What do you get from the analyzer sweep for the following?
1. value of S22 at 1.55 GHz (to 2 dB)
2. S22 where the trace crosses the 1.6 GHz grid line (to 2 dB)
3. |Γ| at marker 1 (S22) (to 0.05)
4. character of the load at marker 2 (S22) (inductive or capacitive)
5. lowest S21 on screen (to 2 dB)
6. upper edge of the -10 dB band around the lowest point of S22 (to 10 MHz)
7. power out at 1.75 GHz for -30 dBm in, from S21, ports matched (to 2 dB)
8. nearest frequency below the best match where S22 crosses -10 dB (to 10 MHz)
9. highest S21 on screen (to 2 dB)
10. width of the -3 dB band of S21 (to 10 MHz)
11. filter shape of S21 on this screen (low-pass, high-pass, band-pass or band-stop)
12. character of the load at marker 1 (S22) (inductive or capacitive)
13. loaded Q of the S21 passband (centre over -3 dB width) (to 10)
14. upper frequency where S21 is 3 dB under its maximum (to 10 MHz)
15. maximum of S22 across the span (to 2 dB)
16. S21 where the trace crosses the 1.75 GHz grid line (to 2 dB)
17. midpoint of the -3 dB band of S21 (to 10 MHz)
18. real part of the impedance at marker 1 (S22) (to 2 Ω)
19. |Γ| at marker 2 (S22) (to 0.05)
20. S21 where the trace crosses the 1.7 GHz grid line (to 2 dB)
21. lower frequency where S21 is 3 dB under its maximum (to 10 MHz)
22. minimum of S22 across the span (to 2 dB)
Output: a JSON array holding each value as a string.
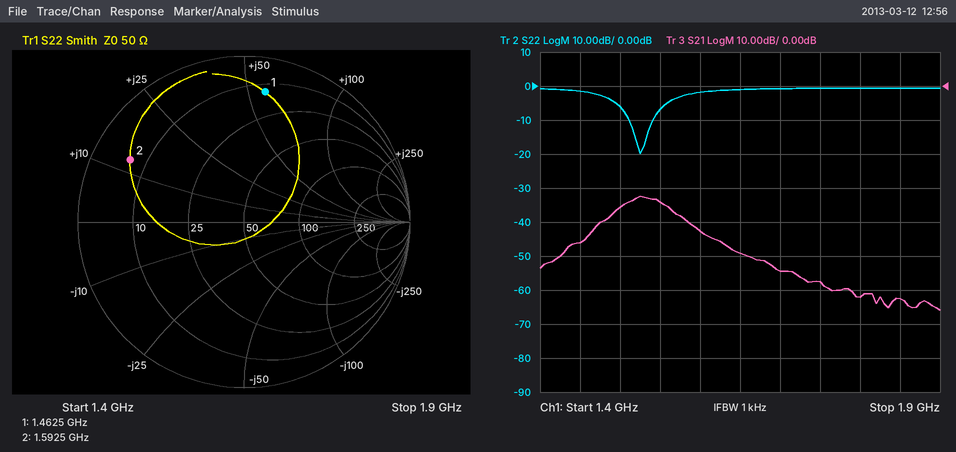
["-6 dB", "-2 dB", "0.80", "inductive", "-66 dB", "1.54 GHz", "-88 dBm", "1.51 GHz", "-32 dB", "60 MHz", "band-pass", "inductive", "30", "1.56 GHz", "0 dB", "-58 dB", "1.53 GHz", "14 Ω", "0.80", "-54 dB", "1.50 GHz", "-20 dB"]
